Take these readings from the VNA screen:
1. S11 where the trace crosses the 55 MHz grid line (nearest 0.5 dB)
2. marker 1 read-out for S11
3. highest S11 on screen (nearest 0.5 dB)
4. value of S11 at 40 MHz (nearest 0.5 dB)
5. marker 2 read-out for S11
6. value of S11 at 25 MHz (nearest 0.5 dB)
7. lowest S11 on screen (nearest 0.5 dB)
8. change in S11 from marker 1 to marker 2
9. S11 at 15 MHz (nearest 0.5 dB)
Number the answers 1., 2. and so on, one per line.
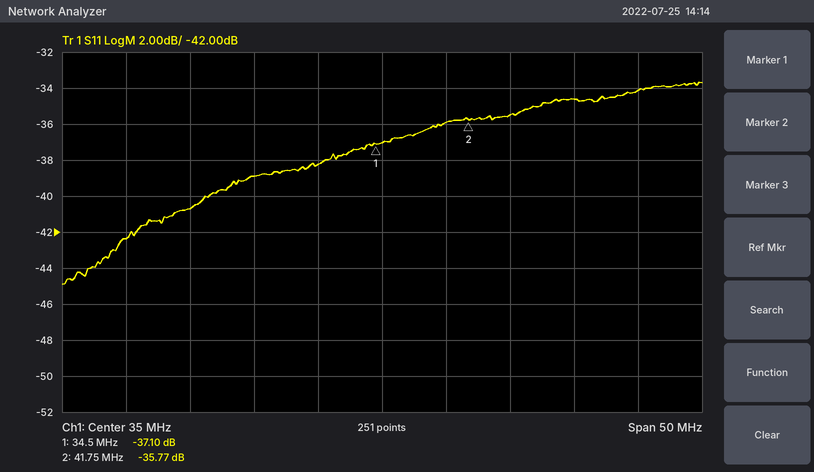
1. -34.0 dB
2. -37.10 dB
3. -33.5 dB
4. -36.0 dB
5. -35.77 dB
6. -39.0 dB
7. -45.0 dB
8. 1.33 dB
9. -42.5 dB
